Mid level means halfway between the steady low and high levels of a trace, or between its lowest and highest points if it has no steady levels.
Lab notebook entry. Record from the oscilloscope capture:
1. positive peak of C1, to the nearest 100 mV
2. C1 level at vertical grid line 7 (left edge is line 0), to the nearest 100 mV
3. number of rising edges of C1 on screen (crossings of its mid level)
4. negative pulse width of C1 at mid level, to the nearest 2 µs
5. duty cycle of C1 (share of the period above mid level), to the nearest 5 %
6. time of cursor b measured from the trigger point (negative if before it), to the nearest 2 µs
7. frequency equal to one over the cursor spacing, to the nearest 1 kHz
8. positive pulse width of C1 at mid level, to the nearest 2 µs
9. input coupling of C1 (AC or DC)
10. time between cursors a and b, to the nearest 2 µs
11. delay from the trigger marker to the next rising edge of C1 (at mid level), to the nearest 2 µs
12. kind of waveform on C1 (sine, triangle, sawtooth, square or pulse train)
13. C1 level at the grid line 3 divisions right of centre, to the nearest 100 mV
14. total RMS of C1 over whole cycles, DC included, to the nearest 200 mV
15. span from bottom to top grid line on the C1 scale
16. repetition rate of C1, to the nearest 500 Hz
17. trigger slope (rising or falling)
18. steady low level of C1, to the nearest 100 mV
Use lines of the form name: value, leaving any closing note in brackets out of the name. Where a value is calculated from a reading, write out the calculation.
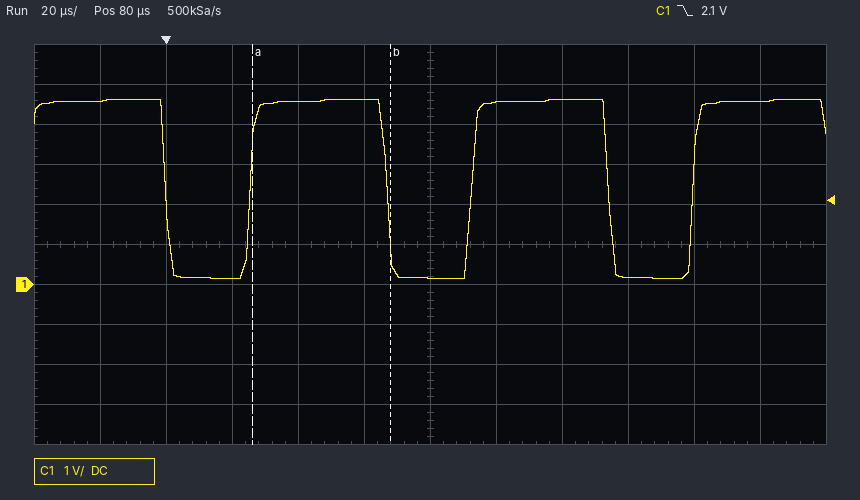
positive peak of C1, to the nearest 100 mV: 4.6 V
C1 level at vertical grid line 7 (left edge is line 0), to the nearest 100 mV: 4.6 V
number of rising edges of C1 on screen: 3
negative pulse width of C1 at mid level, to the nearest 2 µs: 26 µs
duty cycle of C1 (share of the period above mid level), to the nearest 5 %: 60 %
time of cursor b measured from the trigger point (negative if before it), to the nearest 2 µs: +68 µs
frequency equal to one over the cursor spacing, to the nearest 1 kHz: 1 / 42 µs ≈ 24 kHz
positive pulse width of C1 at mid level, to the nearest 2 µs: 42 µs
input coupling of C1: DC
time between cursors a and b, to the nearest 2 µs: 42 µs
delay from the trigger marker to the next rising edge of C1 (at mid level), to the nearest 2 µs: 26 µs
kind of waveform on C1: pulse train
C1 level at the grid line 3 divisions right of centre, to the nearest 100 mV: 200 mV
total RMS of C1 over whole cycles, DC included, to the nearest 200 mV: √(0.6 × (4.6 V)² + 0.4 × (200 mV)²) ≈ 3.6 V
span from bottom to top grid line on the C1 scale: 10 V
repetition rate of C1, to the nearest 500 Hz: 15.0 kHz
trigger slope: falling
steady low level of C1, to the nearest 100 mV: 200 mV
